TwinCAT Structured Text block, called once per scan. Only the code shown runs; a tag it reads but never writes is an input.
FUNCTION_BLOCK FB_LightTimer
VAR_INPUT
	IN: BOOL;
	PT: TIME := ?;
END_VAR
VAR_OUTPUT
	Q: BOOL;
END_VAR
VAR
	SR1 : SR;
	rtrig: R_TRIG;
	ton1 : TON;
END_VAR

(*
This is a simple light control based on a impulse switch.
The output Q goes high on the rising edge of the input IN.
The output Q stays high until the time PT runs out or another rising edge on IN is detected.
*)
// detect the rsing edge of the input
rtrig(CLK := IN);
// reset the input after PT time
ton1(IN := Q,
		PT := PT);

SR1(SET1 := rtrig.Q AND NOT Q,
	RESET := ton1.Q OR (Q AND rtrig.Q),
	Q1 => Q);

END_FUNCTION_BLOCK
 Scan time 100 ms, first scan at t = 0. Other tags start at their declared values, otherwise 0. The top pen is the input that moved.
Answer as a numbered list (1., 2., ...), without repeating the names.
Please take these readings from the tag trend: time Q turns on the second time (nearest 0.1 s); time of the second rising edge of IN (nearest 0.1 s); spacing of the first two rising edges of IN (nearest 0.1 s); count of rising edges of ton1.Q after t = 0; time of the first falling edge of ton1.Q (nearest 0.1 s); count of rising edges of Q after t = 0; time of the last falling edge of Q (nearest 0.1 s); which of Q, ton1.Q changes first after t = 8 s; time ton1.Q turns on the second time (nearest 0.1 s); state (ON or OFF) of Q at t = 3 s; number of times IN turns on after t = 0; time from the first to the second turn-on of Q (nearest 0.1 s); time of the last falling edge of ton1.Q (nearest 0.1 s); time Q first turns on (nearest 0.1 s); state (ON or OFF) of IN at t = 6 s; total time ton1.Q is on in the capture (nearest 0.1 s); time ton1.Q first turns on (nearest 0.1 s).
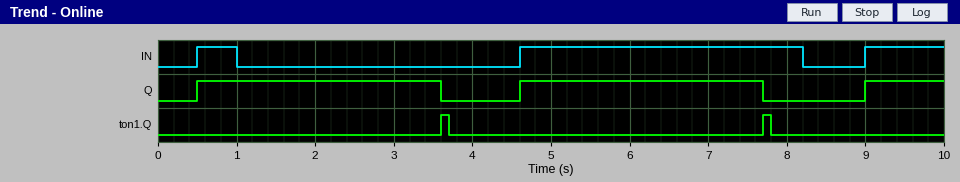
1. 4.6 s
2. 4.6 s
3. 4.1 s
4. 2
5. 3.7 s
6. 3
7. 7.7 s
8. Q
9. 7.7 s
10. ON
11. 3
12. 4.1 s
13. 7.8 s
14. 0.5 s
15. ON
16. 0.2 s
17. 3.6 s
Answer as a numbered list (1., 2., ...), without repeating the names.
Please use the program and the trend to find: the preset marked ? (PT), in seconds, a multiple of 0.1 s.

1. 3.0 s
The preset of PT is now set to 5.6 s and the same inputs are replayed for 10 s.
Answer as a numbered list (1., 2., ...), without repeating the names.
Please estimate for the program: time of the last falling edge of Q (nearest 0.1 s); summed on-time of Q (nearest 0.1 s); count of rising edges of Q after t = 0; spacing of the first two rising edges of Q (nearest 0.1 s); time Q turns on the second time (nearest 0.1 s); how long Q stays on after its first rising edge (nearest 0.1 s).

1. 4.6 s
2. 5.1 s
3. 2
4. 8.5 s
5. 9.0 s
6. 4.1 s
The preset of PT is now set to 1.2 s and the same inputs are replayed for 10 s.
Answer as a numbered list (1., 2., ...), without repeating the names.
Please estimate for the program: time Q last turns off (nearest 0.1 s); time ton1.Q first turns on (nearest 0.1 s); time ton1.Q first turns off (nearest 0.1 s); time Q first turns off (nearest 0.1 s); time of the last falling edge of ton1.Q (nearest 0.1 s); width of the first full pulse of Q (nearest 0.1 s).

1. 5.9 s
2. 1.8 s
3. 1.9 s
4. 1.8 s
5. 6.0 s
6. 1.3 s
